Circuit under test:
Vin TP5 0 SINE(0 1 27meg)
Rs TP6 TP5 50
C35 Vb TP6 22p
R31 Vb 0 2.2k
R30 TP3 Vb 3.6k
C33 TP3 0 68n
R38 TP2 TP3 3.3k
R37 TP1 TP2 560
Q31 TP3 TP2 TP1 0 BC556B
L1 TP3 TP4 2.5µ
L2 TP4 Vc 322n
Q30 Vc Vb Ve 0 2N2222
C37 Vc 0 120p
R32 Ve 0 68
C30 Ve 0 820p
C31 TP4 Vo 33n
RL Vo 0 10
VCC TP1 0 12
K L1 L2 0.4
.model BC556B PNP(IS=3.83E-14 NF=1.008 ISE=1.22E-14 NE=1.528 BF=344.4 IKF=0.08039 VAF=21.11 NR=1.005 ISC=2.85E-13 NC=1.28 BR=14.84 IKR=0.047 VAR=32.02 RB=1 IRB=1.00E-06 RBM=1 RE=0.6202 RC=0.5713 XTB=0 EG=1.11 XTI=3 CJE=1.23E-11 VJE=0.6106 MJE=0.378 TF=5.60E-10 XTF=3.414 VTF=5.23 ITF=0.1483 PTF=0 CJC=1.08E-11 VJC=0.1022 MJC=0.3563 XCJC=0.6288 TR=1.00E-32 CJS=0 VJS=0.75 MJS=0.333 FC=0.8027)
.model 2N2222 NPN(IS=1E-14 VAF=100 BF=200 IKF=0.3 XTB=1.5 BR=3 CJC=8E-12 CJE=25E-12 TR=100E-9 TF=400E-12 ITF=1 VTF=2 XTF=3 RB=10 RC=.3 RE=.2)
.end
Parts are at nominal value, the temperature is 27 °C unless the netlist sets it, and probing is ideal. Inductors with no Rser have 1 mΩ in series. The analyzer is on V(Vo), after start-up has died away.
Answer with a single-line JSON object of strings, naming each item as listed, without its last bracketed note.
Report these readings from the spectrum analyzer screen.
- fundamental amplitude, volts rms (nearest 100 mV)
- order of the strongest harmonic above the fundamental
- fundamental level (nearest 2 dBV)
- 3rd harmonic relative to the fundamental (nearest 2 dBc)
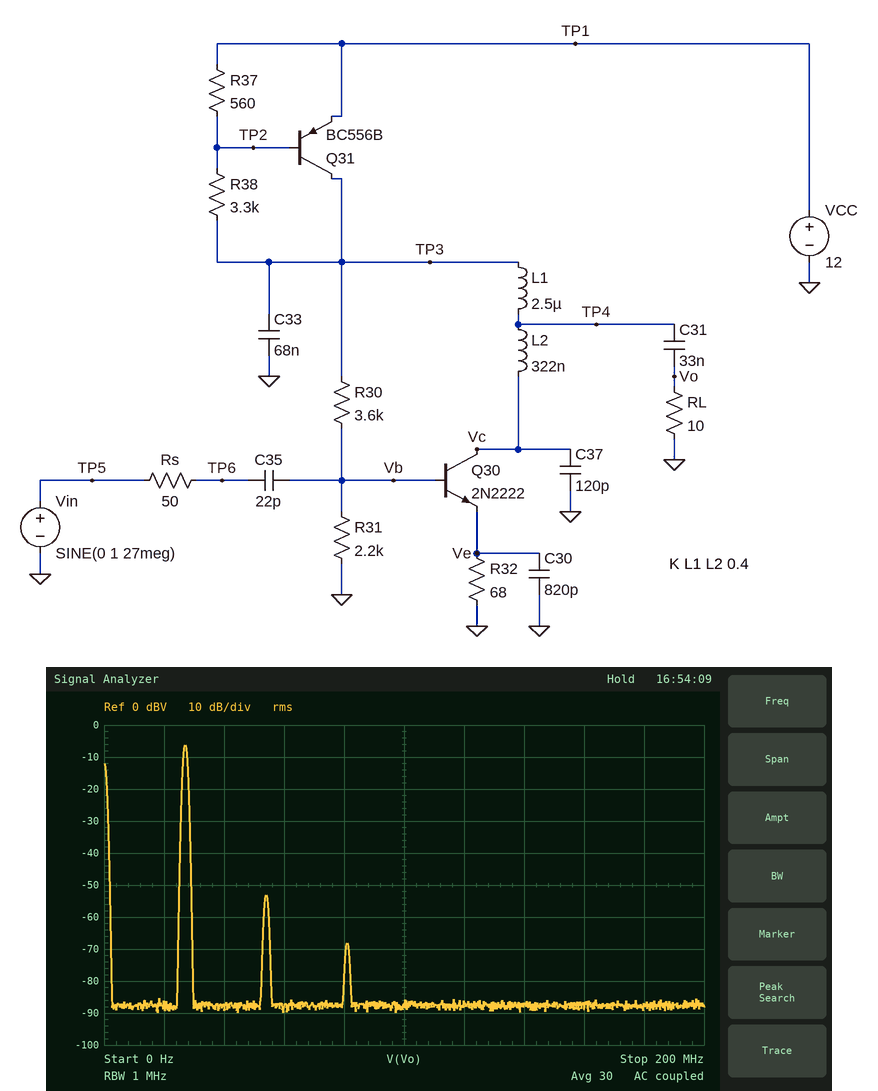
{"fundamental amplitude, volts rms": "500 mV", "order of the strongest harmonic above the fundamental": "2", "fundamental level": "-6 dBV", "3rd harmonic relative to the fundamental": "-62 dBc"}
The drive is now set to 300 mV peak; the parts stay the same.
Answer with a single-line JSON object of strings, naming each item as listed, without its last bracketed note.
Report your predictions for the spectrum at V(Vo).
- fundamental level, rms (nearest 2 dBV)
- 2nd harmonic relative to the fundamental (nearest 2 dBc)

{"fundamental level, rms": "-16 dBV", "2nd harmonic relative to the fundamental": "-56 dBc"}
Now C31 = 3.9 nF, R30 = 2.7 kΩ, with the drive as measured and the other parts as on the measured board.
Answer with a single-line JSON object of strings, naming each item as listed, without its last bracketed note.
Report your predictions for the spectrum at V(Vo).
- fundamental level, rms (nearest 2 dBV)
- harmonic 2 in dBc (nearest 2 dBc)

{"fundamental level, rms": "-6 dBV", "harmonic 2 in dBc": "-44 dBc"}
